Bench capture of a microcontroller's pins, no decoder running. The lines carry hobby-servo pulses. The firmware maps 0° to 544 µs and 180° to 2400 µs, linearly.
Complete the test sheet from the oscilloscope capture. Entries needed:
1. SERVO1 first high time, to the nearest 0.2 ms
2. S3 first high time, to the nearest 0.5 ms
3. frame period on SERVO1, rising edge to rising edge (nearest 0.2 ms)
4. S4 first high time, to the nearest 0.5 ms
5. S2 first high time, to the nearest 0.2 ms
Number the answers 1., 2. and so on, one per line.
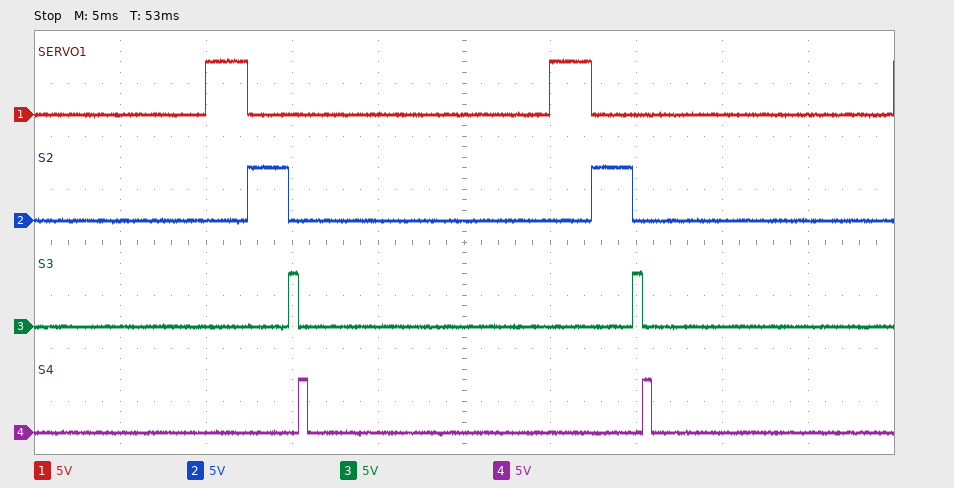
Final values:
1. 2.4 ms
2. 0.5 ms
3. 20.0 ms
4. 0.5 ms
5. 2.4 ms
